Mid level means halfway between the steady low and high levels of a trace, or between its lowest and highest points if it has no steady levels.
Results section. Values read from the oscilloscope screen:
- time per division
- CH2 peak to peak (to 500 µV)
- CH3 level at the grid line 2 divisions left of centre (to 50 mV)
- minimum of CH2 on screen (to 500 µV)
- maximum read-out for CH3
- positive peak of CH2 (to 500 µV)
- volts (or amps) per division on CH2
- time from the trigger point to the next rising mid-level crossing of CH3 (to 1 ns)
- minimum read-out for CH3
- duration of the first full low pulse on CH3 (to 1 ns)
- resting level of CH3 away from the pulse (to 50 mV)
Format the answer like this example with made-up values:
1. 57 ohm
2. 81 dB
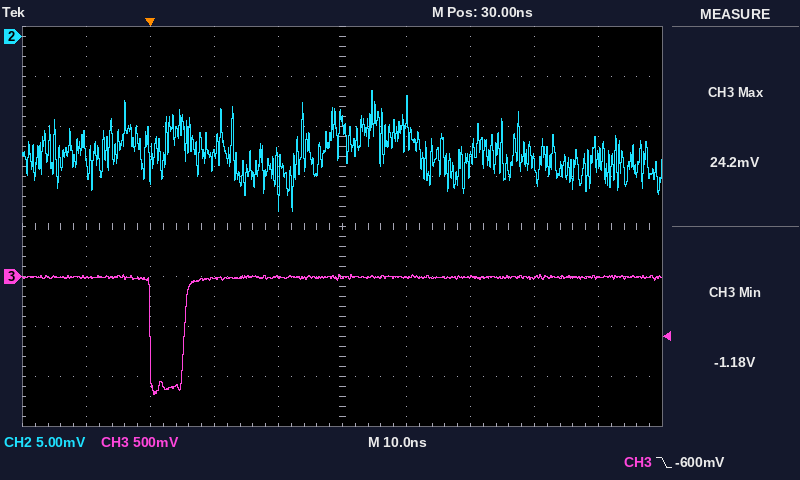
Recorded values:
1. 10 ns
2. 12.0 mV
3. 0 mV
4. -17.5 mV
5. 24.2 mV
6. -5.5 mV
7. 5 mV
8. 5 ns
9. -1.18 V
10. 5 ns
11. 0 mV
